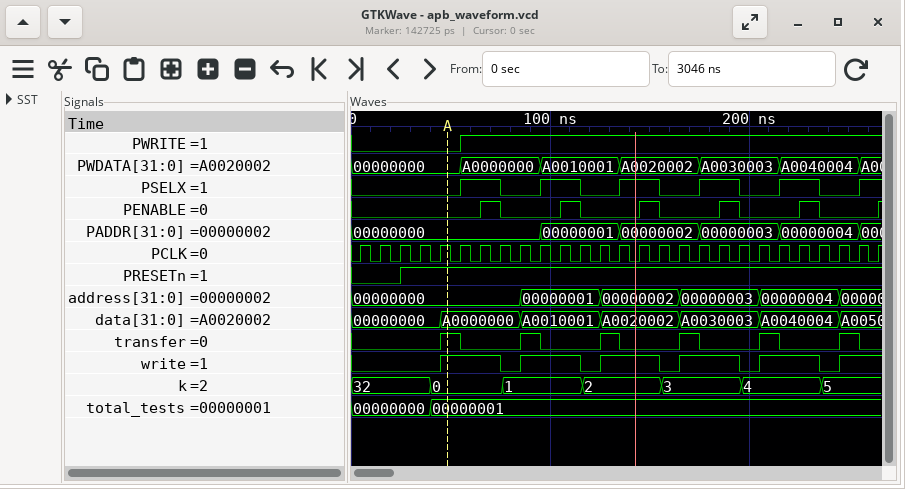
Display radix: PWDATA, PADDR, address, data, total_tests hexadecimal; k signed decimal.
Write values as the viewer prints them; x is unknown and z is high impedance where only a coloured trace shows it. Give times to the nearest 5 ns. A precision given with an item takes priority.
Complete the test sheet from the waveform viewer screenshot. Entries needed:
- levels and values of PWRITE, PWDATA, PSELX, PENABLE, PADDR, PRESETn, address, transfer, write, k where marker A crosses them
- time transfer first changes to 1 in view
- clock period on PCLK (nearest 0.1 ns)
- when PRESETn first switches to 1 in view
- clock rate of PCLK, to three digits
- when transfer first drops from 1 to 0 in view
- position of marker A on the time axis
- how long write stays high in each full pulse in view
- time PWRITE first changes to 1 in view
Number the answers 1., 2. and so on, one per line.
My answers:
1. PWRITE=0, PWDATA=00000000, PSELX=0, PENABLE=0, PADDR=00000000, PRESETn=1, address=00000000, transfer=1, write=1, k=0
2. 45 ns
3. 10 ns
4. 25 ns
5. 100 MHz
6. 55 ns
7. 50 ns
8. 30 ns, 30 ns, 30 ns, 30 ns, 30 ns
9. 55 ns
